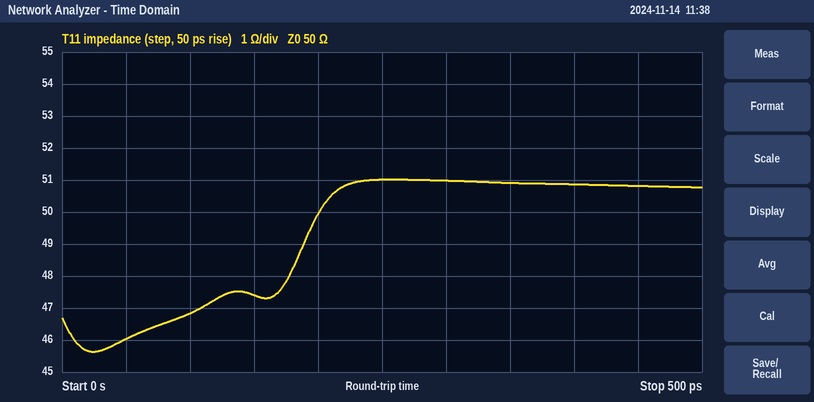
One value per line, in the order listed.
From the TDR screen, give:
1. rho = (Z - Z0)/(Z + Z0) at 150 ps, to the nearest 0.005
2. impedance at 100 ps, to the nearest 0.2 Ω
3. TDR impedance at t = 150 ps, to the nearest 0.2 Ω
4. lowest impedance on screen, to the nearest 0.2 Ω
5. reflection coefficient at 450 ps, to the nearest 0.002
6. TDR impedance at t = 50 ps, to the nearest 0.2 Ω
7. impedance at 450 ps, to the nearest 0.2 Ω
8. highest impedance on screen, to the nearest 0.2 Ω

-0.025
46.8 Ω
47.4 Ω
45.6 Ω
+0.008
46.0 Ω
50.8 Ω
51.0 Ω
